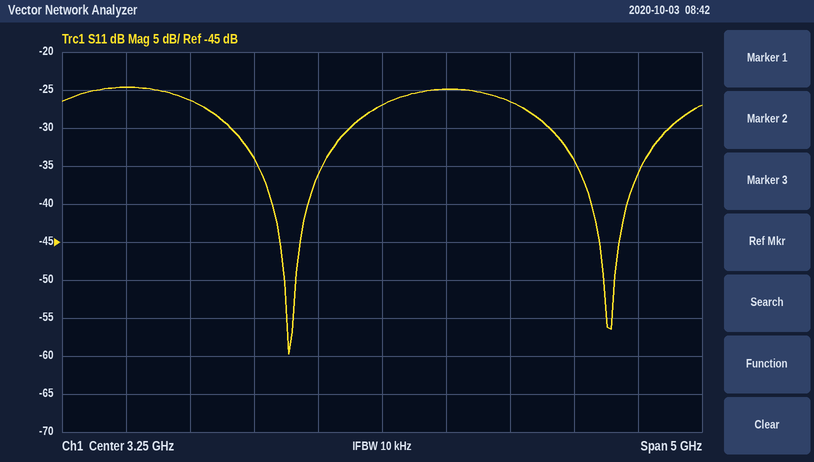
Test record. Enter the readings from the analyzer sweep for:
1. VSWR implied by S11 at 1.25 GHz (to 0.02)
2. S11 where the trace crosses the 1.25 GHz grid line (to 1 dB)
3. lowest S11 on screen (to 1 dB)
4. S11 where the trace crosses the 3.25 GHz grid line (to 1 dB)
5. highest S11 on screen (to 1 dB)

1.12
-25 dB
-60 dB
-27 dB
-25 dB
